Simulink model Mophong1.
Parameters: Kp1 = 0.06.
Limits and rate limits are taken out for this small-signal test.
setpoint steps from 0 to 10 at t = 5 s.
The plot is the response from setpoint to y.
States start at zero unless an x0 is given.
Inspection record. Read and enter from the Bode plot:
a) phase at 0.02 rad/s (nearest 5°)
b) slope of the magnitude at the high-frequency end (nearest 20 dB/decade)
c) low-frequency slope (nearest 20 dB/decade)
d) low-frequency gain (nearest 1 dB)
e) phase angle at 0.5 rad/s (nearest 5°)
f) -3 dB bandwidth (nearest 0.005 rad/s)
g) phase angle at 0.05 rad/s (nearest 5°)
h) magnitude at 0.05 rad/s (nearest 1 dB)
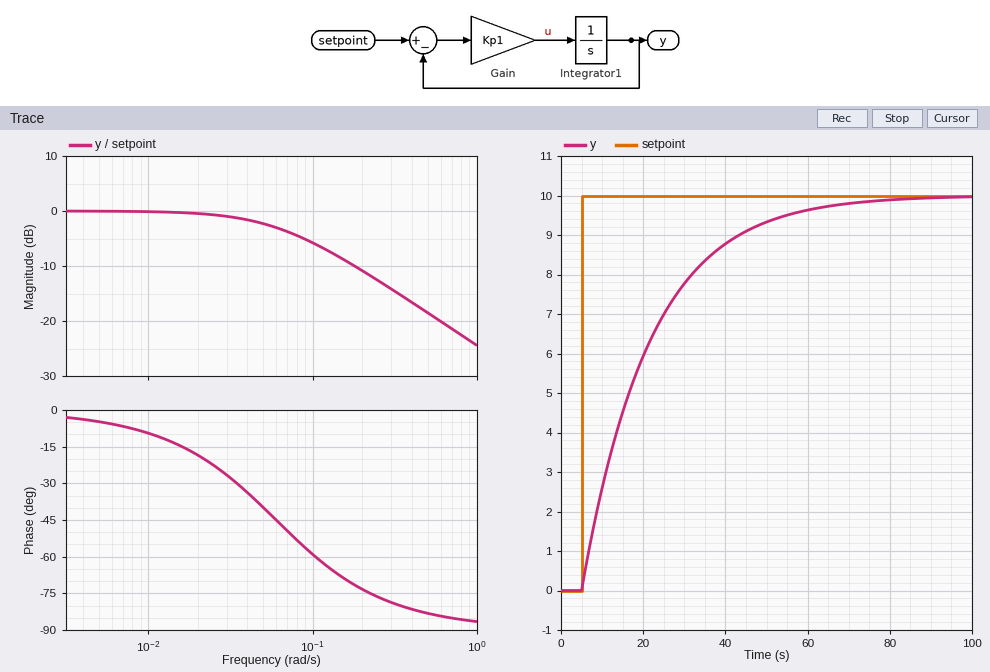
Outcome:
-20°
-20 dB/decade
0 dB/decade
0 dB
-85°
0.060 rad/s
-40°
-2 dB
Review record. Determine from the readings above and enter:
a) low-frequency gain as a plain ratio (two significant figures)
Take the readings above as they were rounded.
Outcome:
1.0
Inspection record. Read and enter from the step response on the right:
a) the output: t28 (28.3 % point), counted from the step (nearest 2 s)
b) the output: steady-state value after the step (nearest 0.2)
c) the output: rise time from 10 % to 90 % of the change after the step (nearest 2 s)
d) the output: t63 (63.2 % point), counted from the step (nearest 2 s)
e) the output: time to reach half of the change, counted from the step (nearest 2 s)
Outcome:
6 s
10.0
36 s
16 s
12 s
